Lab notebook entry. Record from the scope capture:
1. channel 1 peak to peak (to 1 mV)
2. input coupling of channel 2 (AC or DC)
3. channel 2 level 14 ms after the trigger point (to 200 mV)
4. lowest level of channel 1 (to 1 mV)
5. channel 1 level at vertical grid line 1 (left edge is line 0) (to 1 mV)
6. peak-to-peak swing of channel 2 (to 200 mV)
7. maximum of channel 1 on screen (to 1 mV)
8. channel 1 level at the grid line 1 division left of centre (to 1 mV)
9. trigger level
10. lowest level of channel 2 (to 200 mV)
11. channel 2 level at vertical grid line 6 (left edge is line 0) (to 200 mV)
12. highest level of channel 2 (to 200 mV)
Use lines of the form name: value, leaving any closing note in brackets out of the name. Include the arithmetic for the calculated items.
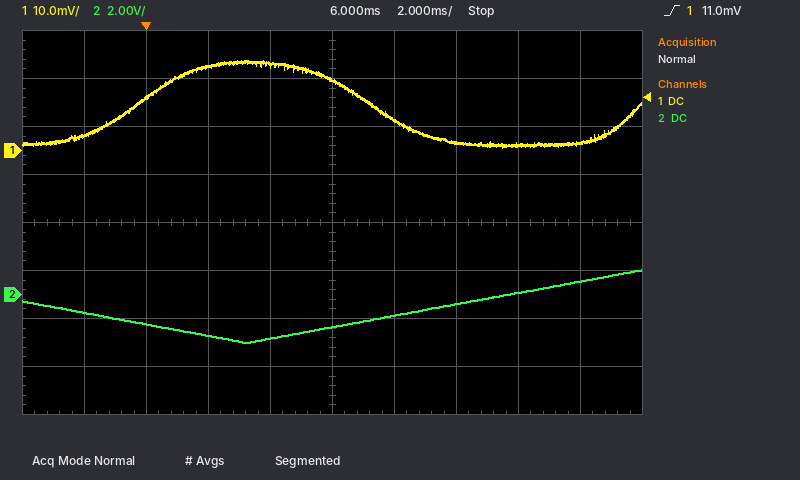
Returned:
channel 1 peak to peak: 19 mV − (1 mV) = 18 mV
input coupling of channel 2: DC
channel 2 level 14 ms after the trigger point: 600 mV
lowest level of channel 1: 1 mV
channel 1 level at vertical grid line 1 (left edge is line 0): 3 mV
peak-to-peak swing of channel 2: 1.0 V − (-2.0 V) = 3.0 V
maximum of channel 1 on screen: 19 mV
channel 1 level at the grid line 1 division left of centre: 18 mV
trigger level: 11.0 mV
lowest level of channel 2: -2.0 V
channel 2 level at vertical grid line 6 (left edge is line 0): -800 mV
highest level of channel 2: 1.0 V
